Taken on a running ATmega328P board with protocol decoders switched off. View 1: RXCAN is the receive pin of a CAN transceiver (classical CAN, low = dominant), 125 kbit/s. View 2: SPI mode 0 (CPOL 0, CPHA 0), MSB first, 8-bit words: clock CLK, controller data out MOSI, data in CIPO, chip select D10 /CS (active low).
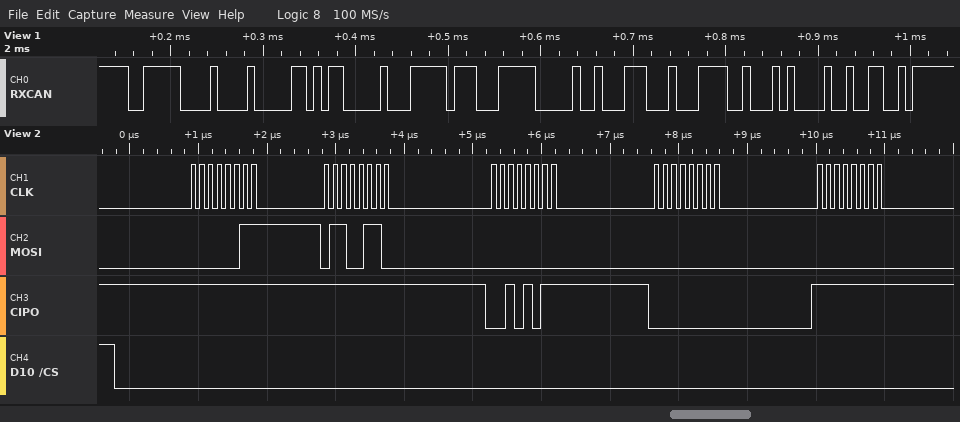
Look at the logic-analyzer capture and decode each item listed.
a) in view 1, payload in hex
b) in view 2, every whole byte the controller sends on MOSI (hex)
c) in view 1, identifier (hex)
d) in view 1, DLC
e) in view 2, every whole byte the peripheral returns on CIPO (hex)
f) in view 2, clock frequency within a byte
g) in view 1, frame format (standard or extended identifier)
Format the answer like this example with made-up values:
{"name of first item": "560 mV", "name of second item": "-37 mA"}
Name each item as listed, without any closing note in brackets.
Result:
{"in view 1, payload in hex": "2B 00 FF 1F 02 38 8F 22", "in view 2, every whole byte the controller sends on MOSI": "03 66 00 00 00", "in view 1, identifier": "0x3E2", "in view 1, DLC": "8", "in view 2, every whole byte the peripheral returns on CIPO": "FF FF 2B 00 FF", "in view 2, clock frequency within a byte": "8 MHz", "in view 1, frame format": "standard"}
